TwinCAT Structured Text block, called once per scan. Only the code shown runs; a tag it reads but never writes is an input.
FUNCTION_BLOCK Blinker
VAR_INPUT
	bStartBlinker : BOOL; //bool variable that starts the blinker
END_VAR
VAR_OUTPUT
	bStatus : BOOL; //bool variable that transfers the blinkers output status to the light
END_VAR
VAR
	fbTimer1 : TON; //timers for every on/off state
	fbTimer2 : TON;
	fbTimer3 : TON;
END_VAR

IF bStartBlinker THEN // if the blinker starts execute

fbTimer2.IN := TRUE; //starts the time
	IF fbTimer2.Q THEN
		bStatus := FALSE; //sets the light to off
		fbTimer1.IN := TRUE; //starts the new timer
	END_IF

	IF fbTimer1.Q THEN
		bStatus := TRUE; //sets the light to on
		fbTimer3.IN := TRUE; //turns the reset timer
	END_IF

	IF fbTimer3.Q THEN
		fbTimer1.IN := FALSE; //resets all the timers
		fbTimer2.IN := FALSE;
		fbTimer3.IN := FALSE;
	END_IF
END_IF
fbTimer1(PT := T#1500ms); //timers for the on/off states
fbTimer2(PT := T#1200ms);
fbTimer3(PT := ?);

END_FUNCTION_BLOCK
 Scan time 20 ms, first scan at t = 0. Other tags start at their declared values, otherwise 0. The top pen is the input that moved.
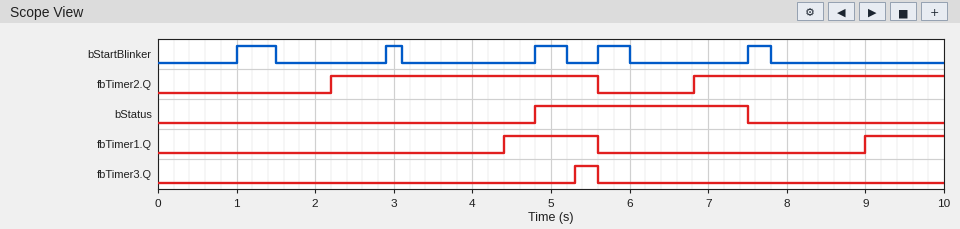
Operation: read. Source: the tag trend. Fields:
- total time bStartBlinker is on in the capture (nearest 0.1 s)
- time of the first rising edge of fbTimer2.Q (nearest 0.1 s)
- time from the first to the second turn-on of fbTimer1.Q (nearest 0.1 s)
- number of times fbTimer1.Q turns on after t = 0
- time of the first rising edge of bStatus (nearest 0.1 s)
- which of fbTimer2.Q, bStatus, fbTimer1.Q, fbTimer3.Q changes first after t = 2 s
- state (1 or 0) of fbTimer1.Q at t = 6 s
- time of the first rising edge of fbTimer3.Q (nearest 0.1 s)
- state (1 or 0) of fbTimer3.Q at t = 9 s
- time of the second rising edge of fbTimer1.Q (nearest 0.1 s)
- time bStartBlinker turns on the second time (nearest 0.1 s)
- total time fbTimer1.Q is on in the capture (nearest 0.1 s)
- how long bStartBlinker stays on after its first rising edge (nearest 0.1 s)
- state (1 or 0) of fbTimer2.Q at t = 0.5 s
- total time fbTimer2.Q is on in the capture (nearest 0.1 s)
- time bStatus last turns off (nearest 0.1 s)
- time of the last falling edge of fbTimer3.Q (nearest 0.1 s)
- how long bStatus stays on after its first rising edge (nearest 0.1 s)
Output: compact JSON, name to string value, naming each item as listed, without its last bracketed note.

{"total time bStartBlinker is on in the capture": "1.8 s", "time of the first rising edge of fbTimer2.Q": "2.2 s", "time from the first to the second turn-on of fbTimer1.Q": "4.6 s", "number of times fbTimer1.Q turns on after t = 0": "2", "time of the first rising edge of bStatus": "4.8 s", "which of fbTimer2.Q, bStatus, fbTimer1.Q, fbTimer3.Q changes first after t = 2 s": "fbTimer2.Q", "state (1 or 0) of fbTimer1.Q at t = 6 s": "0", "time of the first rising edge of fbTimer3.Q": "5.3 s", "state (1 or 0) of fbTimer3.Q at t = 9 s": "0", "time of the second rising edge of fbTimer1.Q": "9.0 s", "time bStartBlinker turns on the second time": "2.9 s", "total time fbTimer1.Q is on in the capture": "2.2 s", "how long bStartBlinker stays on after its first rising edge": "0.5 s", "state (1 or 0) of fbTimer2.Q at t = 0.5 s": "0", "total time fbTimer2.Q is on in the capture": "6.6 s", "time bStatus last turns off": "7.5 s", "time of the last falling edge of fbTimer3.Q": "5.6 s", "how long bStatus stays on after its first rising edge": "2.7 s"}
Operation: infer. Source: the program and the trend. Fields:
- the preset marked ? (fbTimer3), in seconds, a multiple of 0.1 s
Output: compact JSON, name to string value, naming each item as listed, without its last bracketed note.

{"the preset marked ? (fbTimer3), in seconds, a multiple of 0.1 s": "0.5 s"}
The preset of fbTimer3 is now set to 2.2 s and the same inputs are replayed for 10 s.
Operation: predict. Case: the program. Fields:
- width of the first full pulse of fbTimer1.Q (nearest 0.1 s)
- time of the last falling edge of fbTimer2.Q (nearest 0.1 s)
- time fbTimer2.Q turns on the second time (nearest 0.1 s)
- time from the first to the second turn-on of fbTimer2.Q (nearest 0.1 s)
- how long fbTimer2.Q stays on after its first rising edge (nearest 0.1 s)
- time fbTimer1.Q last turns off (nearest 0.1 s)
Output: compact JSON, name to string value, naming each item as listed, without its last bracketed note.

{"width of the first full pulse of fbTimer1.Q": "3.1 s", "time of the last falling edge of fbTimer2.Q": "7.5 s", "time fbTimer2.Q turns on the second time": "8.7 s", "time from the first to the second turn-on of fbTimer2.Q": "6.5 s", "how long fbTimer2.Q stays on after its first rising edge": "5.3 s", "time fbTimer1.Q last turns off": "7.5 s"}
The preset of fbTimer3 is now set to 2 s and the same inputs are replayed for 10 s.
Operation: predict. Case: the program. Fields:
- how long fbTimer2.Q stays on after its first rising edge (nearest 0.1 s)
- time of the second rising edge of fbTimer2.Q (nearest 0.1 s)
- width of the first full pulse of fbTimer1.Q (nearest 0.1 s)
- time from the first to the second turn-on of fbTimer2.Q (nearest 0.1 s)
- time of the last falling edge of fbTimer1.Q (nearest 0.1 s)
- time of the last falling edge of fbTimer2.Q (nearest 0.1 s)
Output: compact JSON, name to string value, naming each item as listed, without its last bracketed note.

{"how long fbTimer2.Q stays on after its first rising edge": "5.3 s", "time of the second rising edge of fbTimer2.Q": "8.7 s", "width of the first full pulse of fbTimer1.Q": "3.1 s", "time from the first to the second turn-on of fbTimer2.Q": "6.5 s", "time of the last falling edge of fbTimer1.Q": "7.5 s", "time of the last falling edge of fbTimer2.Q": "7.5 s"}
